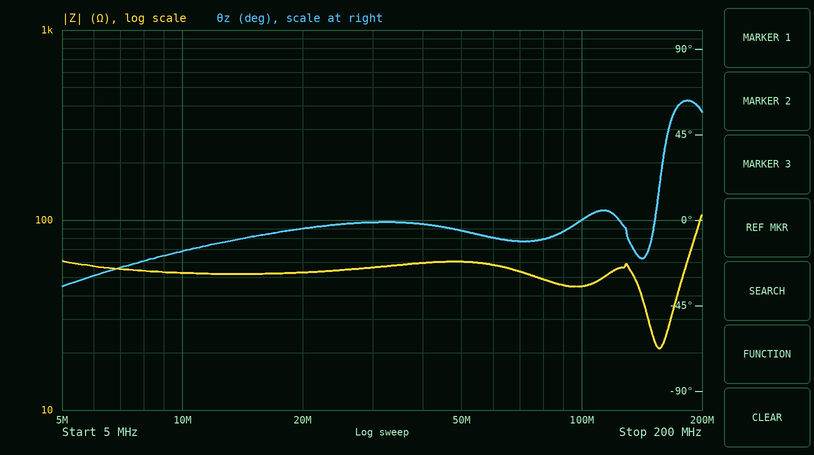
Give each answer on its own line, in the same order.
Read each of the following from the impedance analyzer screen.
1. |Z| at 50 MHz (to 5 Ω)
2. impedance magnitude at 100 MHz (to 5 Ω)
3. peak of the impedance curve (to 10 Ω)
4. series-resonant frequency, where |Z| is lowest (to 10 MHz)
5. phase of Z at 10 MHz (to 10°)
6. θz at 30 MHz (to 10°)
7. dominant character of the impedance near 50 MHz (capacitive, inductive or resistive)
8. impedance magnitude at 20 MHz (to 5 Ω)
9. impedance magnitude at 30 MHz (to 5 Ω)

60 Ω
45 Ω
110 Ω
160 MHz
-20°
0°
resistive
55 Ω
55 Ω
